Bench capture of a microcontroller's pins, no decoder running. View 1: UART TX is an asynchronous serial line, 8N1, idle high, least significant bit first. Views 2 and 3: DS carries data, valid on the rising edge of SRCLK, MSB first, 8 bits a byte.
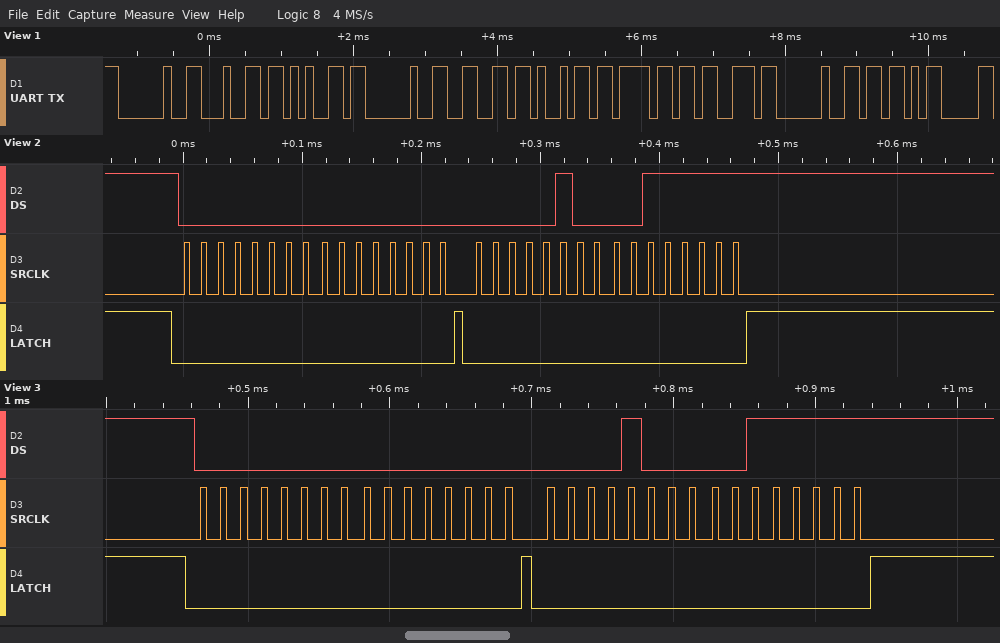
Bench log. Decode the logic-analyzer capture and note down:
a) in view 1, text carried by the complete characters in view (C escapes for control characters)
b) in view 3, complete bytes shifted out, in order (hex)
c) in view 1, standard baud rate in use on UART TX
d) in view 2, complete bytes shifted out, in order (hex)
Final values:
" de fios ["
00 00 08 3F
9600 baud
0x00 0x00 0x04 0x3F
